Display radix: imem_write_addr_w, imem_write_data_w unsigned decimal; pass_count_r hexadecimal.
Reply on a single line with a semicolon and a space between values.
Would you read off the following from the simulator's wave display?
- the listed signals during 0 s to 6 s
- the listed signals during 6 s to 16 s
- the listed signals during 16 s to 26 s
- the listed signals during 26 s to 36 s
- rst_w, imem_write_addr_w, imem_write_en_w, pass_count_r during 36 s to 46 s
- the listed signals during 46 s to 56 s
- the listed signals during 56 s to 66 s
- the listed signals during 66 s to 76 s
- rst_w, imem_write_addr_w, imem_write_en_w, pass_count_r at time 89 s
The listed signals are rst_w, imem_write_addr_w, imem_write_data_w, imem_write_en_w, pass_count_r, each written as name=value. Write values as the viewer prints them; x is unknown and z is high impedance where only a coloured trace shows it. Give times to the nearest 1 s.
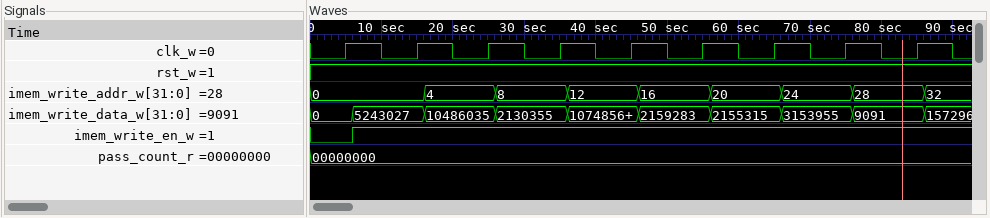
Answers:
rst_w=1, imem_write_addr_w=0, imem_write_data_w=0, imem_write_en_w=0, pass_count_r=00000000; rst_w=1, imem_write_addr_w=0, imem_write_data_w=5243027, imem_write_en_w=1, pass_count_r=00000000; rst_w=1, imem_write_addr_w=4, imem_write_data_w=10486035, imem_write_en_w=1, pass_count_r=00000000; rst_w=1, imem_write_addr_w=8, imem_write_data_w=2130355, imem_write_en_w=1, pass_count_r=00000000; rst_w=1, imem_write_addr_w=12, imem_write_en_w=1, pass_count_r=00000000; rst_w=1, imem_write_addr_w=16, imem_write_data_w=2159283, imem_write_en_w=1, pass_count_r=00000000; rst_w=1, imem_write_addr_w=20, imem_write_data_w=2155315, imem_write_en_w=1, pass_count_r=00000000; rst_w=1, imem_write_addr_w=24, imem_write_data_w=3153955, imem_write_en_w=1, pass_count_r=00000000; rst_w=1, imem_write_addr_w=32, imem_write_en_w=1, pass_count_r=00000000
